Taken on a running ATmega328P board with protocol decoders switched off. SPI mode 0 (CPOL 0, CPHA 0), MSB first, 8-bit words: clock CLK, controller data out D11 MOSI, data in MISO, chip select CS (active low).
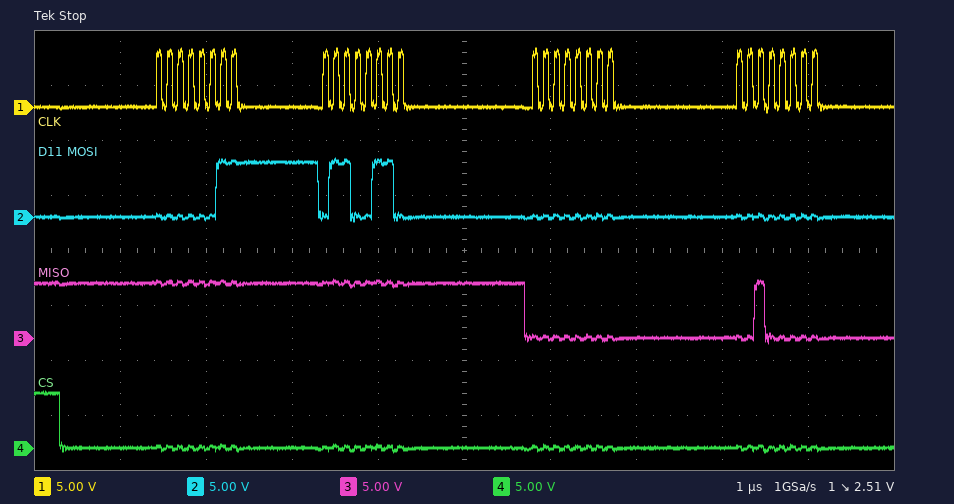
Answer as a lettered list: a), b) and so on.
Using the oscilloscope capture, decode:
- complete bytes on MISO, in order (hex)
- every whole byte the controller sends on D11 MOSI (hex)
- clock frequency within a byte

a) FF FF 00 20
b) 03 66 00 00
c) 8 MHz
